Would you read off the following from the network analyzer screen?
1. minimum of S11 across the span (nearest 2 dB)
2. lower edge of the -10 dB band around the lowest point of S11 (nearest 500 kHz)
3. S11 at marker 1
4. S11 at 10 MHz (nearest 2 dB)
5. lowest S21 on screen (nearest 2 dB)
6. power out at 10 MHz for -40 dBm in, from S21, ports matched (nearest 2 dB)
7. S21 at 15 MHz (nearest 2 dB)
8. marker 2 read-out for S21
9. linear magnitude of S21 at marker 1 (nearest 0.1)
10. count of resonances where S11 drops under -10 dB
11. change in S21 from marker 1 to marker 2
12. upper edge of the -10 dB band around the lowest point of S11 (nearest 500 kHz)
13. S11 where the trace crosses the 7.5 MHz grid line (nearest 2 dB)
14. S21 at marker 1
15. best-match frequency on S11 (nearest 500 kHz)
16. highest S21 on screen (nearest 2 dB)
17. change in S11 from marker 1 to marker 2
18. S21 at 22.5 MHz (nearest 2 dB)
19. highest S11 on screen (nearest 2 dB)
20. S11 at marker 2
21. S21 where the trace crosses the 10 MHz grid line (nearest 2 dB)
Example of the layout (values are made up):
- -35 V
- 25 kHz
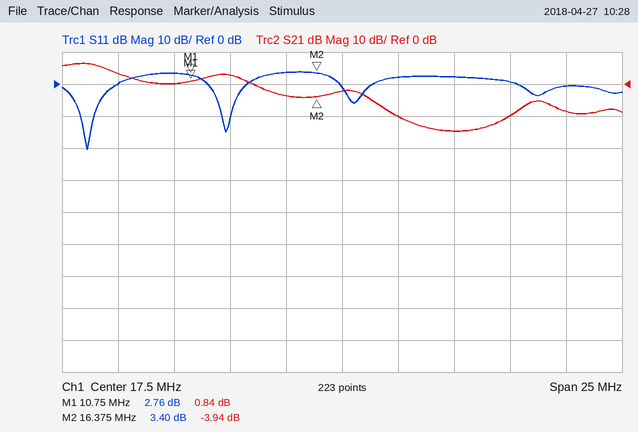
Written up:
- -20 dB
- 6.0 MHz
- 2.76 dB
- 4 dB
- -14 dB
- -40 dBm
- -4 dB
- -3.94 dB
- 1.1
- 2
- -4.78 dB
- 6.5 MHz
- 0 dB
- 0.84 dB
- 6.0 MHz
- 6 dB
- 0.64 dB
- -14 dB
- 4 dB
- 3.40 dB
- 0 dB
